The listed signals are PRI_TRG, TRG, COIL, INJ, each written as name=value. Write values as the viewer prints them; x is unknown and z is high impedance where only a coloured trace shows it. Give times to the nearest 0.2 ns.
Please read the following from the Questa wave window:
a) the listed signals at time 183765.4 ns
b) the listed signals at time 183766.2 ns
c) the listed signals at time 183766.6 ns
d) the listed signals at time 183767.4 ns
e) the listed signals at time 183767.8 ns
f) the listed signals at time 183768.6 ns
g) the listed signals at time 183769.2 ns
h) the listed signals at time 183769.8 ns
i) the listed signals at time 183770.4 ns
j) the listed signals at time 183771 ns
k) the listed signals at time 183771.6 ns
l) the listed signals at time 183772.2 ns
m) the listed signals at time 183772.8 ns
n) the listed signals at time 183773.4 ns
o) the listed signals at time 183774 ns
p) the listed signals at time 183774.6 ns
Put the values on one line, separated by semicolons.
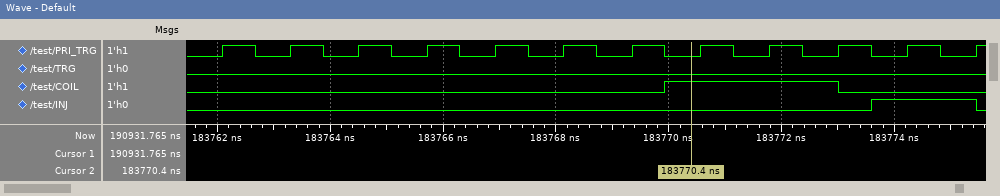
PRI_TRG=0, TRG=0, COIL=0, INJ=0; PRI_TRG=1, TRG=0, COIL=0, INJ=0; PRI_TRG=0, TRG=0, COIL=0, INJ=0; PRI_TRG=1, TRG=0, COIL=0, INJ=0; PRI_TRG=0, TRG=0, COIL=0, INJ=0; PRI_TRG=1, TRG=0, COIL=0, INJ=0; PRI_TRG=0, TRG=0, COIL=0, INJ=0; PRI_TRG=1, TRG=0, COIL=0, INJ=0; PRI_TRG=0, TRG=0, COIL=1, INJ=0; PRI_TRG=1, TRG=0, COIL=1, INJ=0; PRI_TRG=0, TRG=0, COIL=1, INJ=0; PRI_TRG=1, TRG=0, COIL=1, INJ=0; PRI_TRG=0, TRG=0, COIL=1, INJ=0; PRI_TRG=1, TRG=0, COIL=0, INJ=0; PRI_TRG=0, TRG=0, COIL=0, INJ=1; PRI_TRG=1, TRG=0, COIL=0, INJ=1
